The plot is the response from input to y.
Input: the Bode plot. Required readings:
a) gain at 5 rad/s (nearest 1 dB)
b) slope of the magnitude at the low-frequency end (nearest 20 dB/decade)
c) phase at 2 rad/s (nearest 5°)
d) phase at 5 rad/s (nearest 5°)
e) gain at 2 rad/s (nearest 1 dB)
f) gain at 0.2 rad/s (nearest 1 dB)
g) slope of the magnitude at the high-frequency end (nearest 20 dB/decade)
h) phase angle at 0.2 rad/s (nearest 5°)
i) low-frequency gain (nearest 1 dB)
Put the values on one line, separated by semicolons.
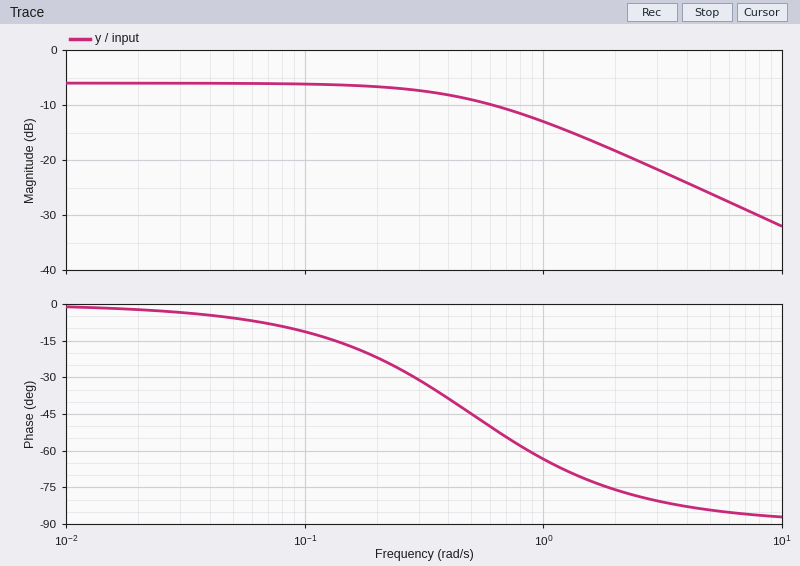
-26 dB; 0 dB/decade; -75°; -85°; -18 dB; -7 dB; -20 dB/decade; -20°; -6 dB
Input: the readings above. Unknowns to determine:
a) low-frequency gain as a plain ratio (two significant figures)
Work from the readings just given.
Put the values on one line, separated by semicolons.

0.50
